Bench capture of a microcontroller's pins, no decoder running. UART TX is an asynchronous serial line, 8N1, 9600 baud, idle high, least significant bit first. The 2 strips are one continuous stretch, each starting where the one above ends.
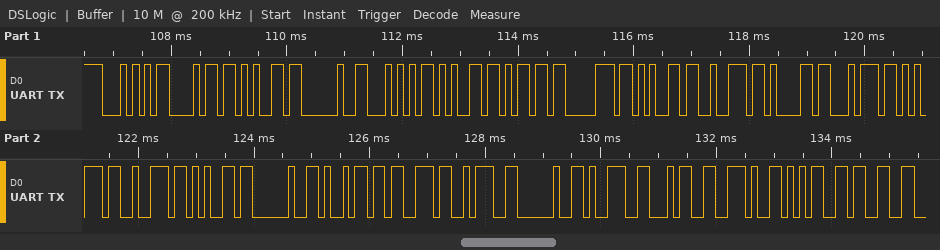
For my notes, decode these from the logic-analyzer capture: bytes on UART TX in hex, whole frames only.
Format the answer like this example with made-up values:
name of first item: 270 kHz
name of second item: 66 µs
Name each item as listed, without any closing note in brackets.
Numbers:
bytes on UART TX in hex, whole frames only: 0x54 0x68 0x65 0x20 0x54 0x65 0x6D 0x70 0x65 0x72 0x61 0x74 0x75 0x72 0x65 0x20 0x69 0x73 0x3A 0x20 0x39 0x34 0x2E 0x35 0x33
